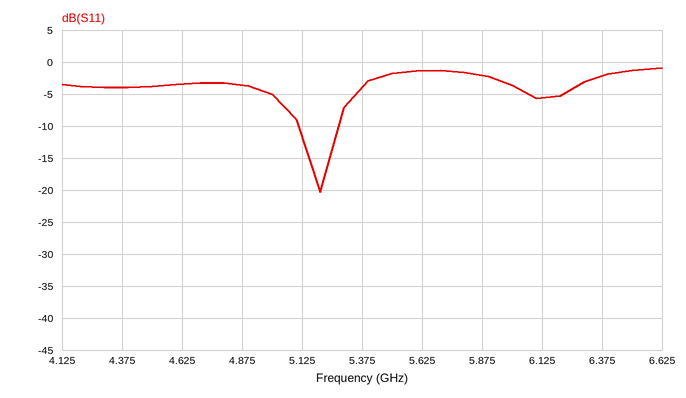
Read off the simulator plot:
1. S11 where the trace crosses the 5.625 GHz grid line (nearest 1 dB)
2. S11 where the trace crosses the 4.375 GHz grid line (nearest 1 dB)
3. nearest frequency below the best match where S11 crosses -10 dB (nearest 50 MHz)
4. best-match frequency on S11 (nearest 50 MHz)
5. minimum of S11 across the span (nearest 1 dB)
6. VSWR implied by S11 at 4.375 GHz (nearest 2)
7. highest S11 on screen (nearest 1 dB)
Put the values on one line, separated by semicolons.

-1 dB; -4 dB; 5.10 GHz; 5.20 GHz; -20 dB; 4; -1 dB
